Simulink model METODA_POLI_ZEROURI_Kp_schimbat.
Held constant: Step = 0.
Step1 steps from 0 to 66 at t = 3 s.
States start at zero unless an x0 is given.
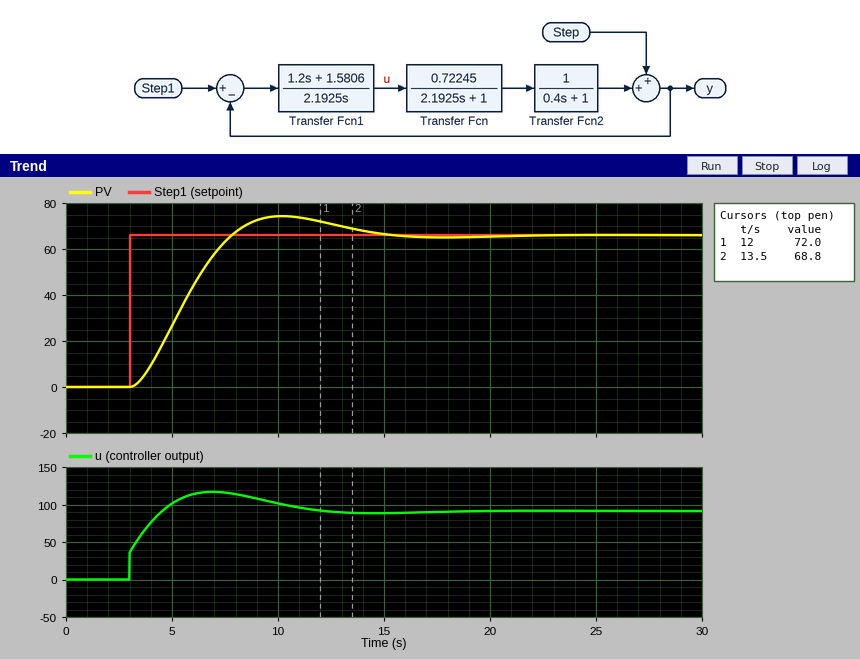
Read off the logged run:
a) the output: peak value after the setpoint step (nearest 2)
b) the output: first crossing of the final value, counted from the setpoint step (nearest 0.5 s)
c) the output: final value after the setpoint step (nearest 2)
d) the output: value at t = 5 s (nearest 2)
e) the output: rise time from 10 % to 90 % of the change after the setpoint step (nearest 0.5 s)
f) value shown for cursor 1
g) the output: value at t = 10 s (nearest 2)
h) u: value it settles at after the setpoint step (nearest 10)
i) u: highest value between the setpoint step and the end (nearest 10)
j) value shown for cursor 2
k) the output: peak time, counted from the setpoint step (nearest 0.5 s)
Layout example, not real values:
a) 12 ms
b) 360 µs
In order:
a) 74
b) 5.0 s
c) 66
d) 26
e) 3.5 s
f) 72.0
g) 74
h) 90
i) 120
j) 68.8
k) 7.0 s
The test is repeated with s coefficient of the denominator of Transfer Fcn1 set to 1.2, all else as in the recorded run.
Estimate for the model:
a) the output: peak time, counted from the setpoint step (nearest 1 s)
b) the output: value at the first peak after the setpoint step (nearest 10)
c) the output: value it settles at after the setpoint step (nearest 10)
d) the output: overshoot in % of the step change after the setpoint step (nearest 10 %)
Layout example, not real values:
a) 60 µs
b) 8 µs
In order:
a) 5 s
b) 80
c) 70
d) 20 %
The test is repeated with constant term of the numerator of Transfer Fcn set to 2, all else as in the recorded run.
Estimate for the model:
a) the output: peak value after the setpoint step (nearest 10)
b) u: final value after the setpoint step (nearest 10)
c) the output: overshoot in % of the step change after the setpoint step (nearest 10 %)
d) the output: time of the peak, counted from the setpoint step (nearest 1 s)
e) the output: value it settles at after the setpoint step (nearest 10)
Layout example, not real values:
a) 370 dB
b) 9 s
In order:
a) 80
b) 30
c) 30 %
d) 4 s
e) 70
